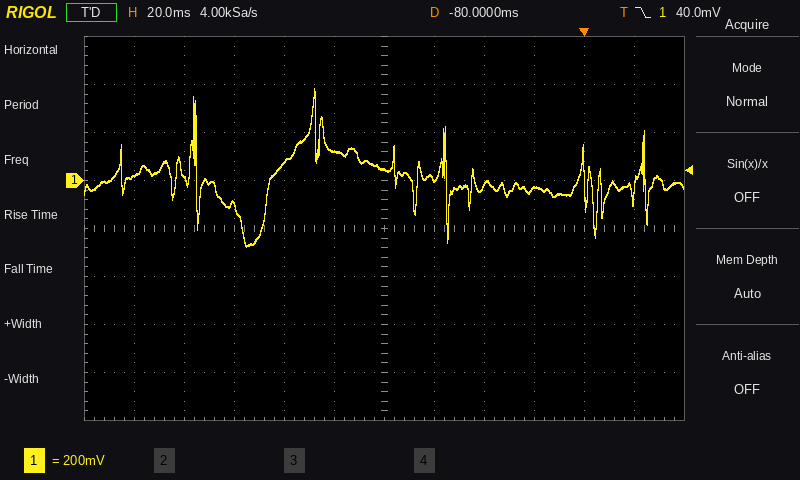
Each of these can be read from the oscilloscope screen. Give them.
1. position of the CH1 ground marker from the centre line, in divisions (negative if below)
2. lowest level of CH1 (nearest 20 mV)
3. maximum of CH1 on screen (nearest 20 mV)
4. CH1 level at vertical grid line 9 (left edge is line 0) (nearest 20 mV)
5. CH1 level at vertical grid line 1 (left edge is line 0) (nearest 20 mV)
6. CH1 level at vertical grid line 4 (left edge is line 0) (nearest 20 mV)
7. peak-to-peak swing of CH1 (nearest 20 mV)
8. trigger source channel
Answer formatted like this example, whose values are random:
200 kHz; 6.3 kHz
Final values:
+1.0 div; -280 mV; 380 mV; -40 mV; 20 mV; 80 mV; 660 mV; CH1
